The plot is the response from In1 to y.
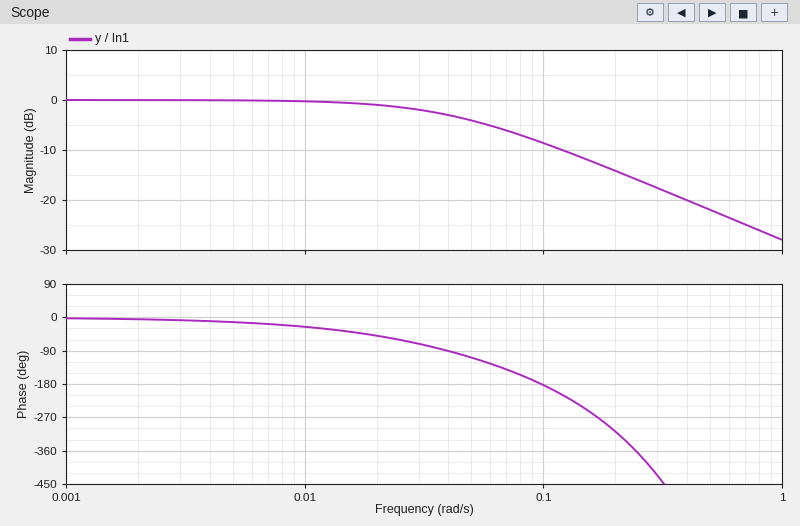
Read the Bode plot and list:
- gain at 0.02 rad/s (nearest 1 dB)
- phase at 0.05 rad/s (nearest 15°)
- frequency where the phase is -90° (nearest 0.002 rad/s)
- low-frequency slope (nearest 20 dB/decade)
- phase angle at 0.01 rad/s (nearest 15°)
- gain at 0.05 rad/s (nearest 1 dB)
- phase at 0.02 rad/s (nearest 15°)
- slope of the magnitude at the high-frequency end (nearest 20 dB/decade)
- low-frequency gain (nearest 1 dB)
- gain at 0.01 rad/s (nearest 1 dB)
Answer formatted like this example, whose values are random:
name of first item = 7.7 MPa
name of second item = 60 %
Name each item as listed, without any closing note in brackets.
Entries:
gain at 0.02 rad/s = -1 dB
phase at 0.05 rad/s = -105°
frequency where the phase is -90° = 0.040 rad/s
low-frequency slope = 0 dB/decade
phase angle at 0.01 rad/s = -30°
gain at 0.05 rad/s = -4 dB
phase at 0.02 rad/s = -45°
slope of the magnitude at the high-frequency end = -20 dB/decade
low-frequency gain = 0 dB
gain at 0.01 rad/s = 0 dB
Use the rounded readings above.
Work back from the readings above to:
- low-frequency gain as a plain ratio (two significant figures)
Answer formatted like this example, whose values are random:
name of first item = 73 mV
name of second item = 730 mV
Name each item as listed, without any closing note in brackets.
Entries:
low-frequency gain as a plain ratio = 1.0
